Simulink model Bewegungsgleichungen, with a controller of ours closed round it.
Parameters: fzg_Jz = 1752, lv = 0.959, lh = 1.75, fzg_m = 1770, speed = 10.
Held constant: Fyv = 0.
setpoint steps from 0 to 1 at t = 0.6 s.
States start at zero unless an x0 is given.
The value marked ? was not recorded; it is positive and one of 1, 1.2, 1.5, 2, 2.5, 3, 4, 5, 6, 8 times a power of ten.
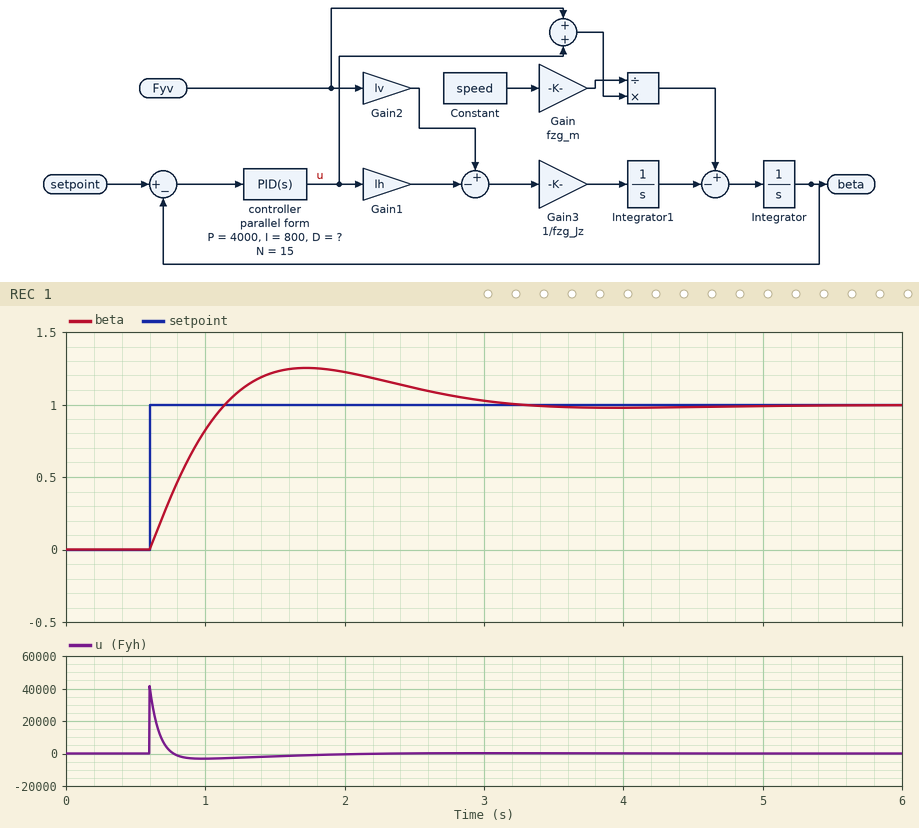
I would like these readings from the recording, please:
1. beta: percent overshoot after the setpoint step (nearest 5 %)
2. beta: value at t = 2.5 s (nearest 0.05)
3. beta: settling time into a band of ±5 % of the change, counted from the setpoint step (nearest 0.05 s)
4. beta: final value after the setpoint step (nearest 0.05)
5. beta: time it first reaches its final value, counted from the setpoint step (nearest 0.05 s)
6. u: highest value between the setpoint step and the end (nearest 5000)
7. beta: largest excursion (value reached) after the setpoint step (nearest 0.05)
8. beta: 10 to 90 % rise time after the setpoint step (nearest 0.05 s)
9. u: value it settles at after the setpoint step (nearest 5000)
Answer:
25 %
1.10
2.25 s
1.00
0.55 s
40000
1.25
0.40 s
0
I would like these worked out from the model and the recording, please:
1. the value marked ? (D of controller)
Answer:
2500
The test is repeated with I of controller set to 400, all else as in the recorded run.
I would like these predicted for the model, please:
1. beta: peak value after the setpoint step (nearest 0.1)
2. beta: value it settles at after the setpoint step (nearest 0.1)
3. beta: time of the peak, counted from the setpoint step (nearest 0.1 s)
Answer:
1.2
1.0
1.1 s
